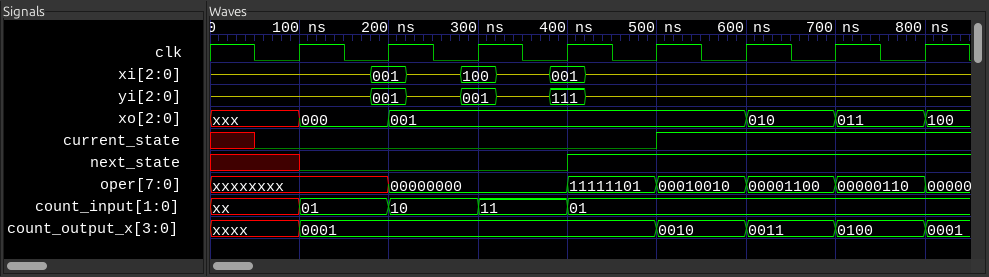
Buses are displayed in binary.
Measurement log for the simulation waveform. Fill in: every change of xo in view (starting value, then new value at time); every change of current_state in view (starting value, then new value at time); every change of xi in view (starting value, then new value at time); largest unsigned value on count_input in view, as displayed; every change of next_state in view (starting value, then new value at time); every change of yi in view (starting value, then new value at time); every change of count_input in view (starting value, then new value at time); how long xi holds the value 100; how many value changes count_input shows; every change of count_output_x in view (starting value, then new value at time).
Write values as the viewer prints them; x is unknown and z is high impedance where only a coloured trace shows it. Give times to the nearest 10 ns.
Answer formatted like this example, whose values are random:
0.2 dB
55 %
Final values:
xxx, 000 at 100 ns, 001 at 200 ns, 010 at 600 ns, 011 at 700 ns, 100 at 800 ns
x, 0 at 50 ns, 1 at 500 ns
z, 001 at 180 ns, z at 220 ns, 100 at 280 ns, z at 320 ns, 001 at 380 ns, z at 420 ns
11
x, 0 at 100 ns, 1 at 400 ns
z, 001 at 180 ns, z at 220 ns, 001 at 280 ns, z at 320 ns, 111 at 380 ns, z at 420 ns
xx, 01 at 100 ns, 10 at 200 ns, 11 at 300 ns, 01 at 400 ns
40 ns
4
xxxx, 0001 at 100 ns, 0010 at 500 ns, 0011 at 600 ns, 0100 at 700 ns, 0001 at 800 ns
